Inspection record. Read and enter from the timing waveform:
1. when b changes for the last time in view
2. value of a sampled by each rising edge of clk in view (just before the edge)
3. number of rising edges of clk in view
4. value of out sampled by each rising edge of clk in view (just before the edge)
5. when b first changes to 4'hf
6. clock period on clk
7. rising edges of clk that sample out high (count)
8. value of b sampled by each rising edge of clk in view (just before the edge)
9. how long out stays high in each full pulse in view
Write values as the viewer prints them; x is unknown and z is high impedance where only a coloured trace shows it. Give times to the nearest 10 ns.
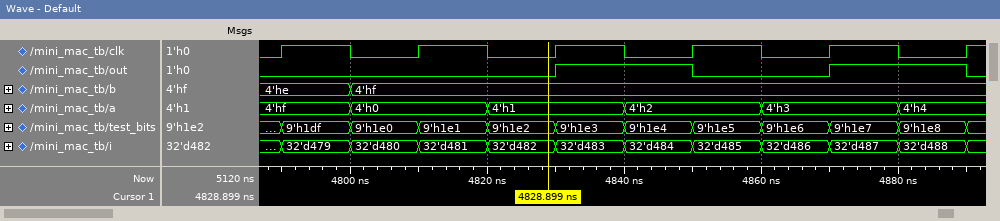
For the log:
4800 ns
4'hf, 4'h0, 4'h1, 4'h2, 4'h3, 4'h4
6
0 0 0 1 0 1
4800 ns
20 ns
2
4'he, 4'hf, 4'hf, 4'hf, 4'hf, 4'hf
20 ns, 20 ns
